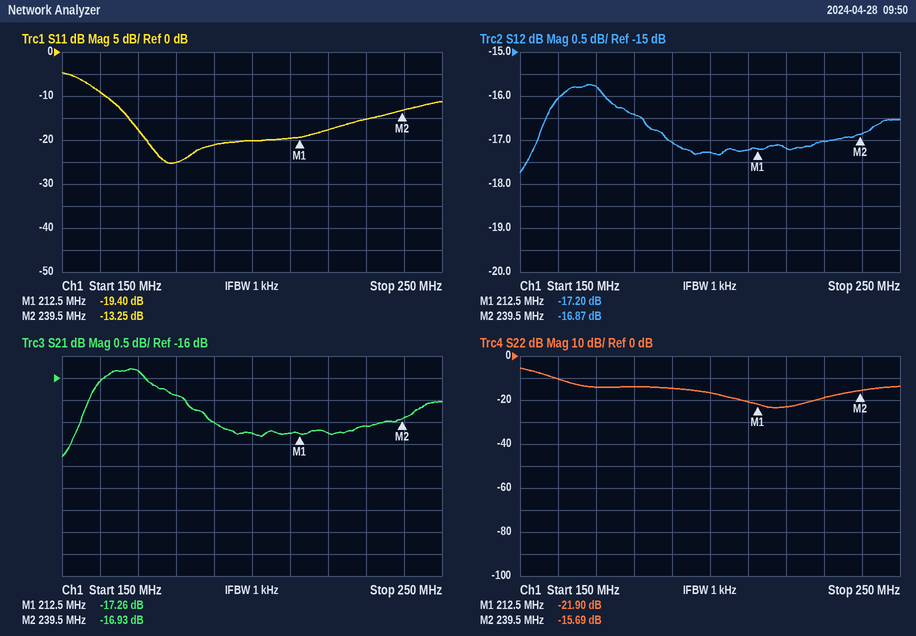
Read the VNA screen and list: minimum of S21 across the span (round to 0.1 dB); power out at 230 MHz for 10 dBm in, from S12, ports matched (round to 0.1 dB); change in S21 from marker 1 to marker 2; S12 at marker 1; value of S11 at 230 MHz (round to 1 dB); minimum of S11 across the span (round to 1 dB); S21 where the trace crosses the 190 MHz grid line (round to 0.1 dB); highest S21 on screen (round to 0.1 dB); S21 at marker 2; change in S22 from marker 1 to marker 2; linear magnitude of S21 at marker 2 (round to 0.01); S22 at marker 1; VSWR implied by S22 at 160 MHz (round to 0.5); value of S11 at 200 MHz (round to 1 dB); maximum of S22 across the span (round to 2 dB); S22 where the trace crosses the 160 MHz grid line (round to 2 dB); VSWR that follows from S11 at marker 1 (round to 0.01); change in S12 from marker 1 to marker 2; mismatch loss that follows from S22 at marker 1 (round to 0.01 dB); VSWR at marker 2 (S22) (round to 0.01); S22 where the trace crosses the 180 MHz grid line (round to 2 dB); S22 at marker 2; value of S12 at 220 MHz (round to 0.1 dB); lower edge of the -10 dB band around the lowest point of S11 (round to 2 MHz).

-17.8 dB
-7.0 dBm
0.33 dB
-17.20 dB
-15 dB
-25 dB
-17.0 dB
-15.8 dB
-16.93 dB
6.21 dB
0.14
-21.90 dB
2.0
-20 dB
-6 dB
-10 dB
1.24
0.33 dB
0.03 dB
1.39
-14 dB
-15.69 dB
-17.2 dB
162 MHz
